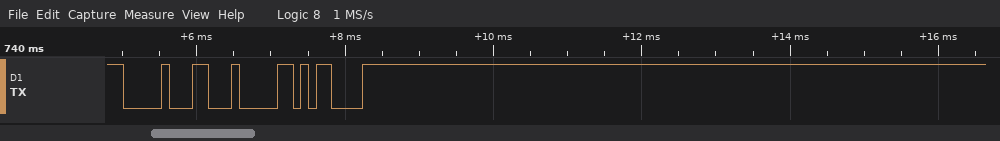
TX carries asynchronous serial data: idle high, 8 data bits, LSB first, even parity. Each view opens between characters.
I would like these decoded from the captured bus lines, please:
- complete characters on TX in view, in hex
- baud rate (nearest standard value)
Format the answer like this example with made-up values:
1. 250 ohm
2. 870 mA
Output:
1. 10, 04, 0D
2. 9600 baud
